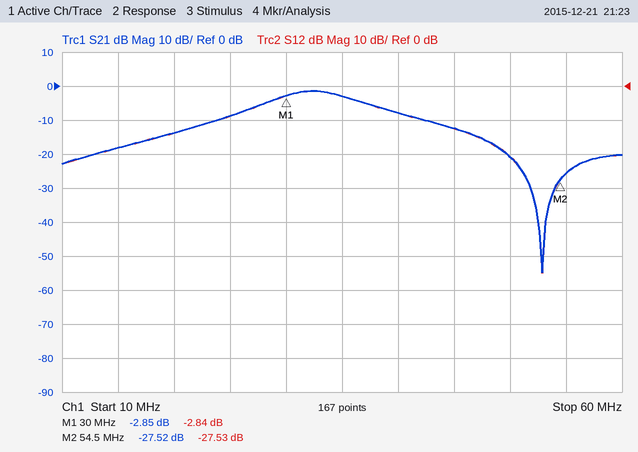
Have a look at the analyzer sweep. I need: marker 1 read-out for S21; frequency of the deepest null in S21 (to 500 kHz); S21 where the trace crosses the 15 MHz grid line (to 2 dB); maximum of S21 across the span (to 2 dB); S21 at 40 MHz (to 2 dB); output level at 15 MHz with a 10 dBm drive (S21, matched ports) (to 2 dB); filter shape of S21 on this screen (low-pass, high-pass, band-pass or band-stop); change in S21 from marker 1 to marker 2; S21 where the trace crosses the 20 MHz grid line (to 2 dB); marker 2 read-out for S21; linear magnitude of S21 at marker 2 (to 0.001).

-2.85 dB
53.0 MHz
-18 dB
-2 dB
-8 dB
-8 dBm
band-pass
-24.67 dB
-14 dB
-27.52 dB
0.042
